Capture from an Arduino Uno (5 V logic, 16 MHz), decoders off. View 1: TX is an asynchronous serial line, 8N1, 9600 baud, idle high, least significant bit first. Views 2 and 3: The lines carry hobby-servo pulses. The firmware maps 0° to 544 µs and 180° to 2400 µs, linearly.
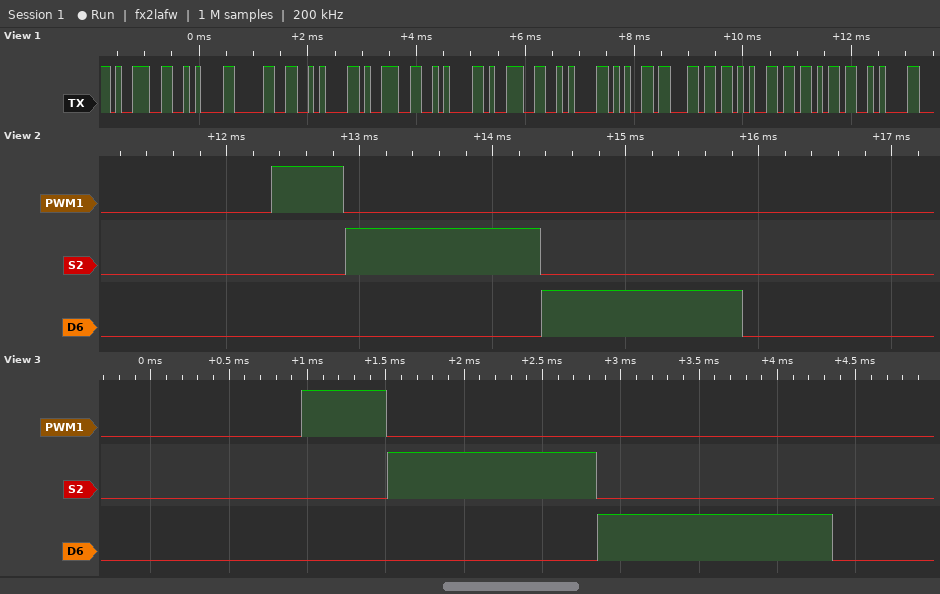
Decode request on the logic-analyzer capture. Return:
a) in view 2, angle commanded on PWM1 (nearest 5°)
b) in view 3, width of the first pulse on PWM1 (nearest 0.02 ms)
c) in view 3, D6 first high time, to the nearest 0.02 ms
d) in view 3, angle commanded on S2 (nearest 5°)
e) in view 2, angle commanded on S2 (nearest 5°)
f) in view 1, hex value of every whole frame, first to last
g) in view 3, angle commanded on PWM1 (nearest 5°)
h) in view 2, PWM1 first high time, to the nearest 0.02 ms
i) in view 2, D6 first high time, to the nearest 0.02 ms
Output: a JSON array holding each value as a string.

["0°", "0.54 ms", "1.50 ms", "75°", "90°", "39 0A 30 0A 39 0A 39 0A 65 6C 65 6B 0A", "0°", "0.54 ms", "1.50 ms"]
